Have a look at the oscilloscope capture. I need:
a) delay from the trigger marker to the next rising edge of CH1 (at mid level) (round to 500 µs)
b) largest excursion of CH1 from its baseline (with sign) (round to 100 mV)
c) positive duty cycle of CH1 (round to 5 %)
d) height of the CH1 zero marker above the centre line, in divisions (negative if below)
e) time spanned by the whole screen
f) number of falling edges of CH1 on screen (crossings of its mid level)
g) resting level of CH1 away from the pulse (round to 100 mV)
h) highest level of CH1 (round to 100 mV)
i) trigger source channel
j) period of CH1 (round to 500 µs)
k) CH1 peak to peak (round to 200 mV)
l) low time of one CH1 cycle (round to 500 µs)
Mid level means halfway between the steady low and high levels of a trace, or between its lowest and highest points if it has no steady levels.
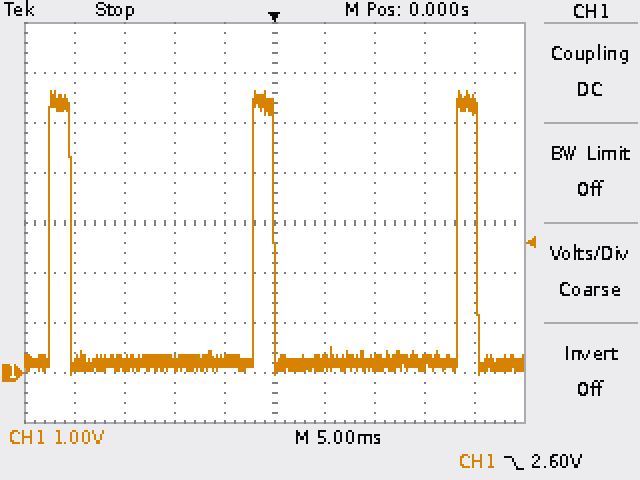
18.5 ms
+5.4 V
10 %
-3.0 div
50 ms
3
200 mV
5.6 V
CH1
20.5 ms
5.6 V
18.5 ms
